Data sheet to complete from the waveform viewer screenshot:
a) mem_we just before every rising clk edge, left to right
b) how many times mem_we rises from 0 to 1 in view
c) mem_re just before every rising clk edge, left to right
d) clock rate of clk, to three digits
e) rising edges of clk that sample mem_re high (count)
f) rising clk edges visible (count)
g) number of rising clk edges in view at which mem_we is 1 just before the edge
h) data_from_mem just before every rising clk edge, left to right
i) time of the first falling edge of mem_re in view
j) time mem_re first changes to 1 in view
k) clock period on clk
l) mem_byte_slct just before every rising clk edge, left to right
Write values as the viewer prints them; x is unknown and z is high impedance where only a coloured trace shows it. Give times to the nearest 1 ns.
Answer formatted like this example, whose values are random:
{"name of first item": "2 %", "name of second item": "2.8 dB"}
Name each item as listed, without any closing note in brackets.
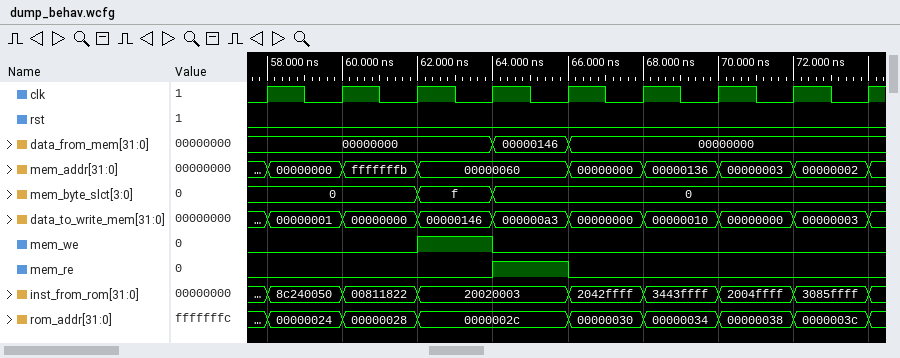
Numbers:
{"mem_we just before every rising clk edge, left to right": "0 0 0 1 0 0 0 0 0", "how many times mem_we rises from 0 to 1 in view": "1", "mem_re just before every rising clk edge, left to right": "0 0 0 0 1 0 0 0 0", "clock rate of clk, to three digits": "500 MHz", "rising edges of clk that sample mem_re high": "1", "rising clk edges visible": "9", "number of rising clk edges in view at which mem_we is 1 just before the edge": "1", "data_from_mem just before every rising clk edge, left to right": "00000000, 00000000, 00000000, 00000000, 00000146, 00000000, 00000000, 00000000, 00000000", "time of the first falling edge of mem_re in view": "66 ns", "time mem_re first changes to 1 in view": "64 ns", "clock period on clk": "2 ns", "mem_byte_slct just before every rising clk edge, left to right": "0, 0, 0, f, 0, 0, 0, 0, 0"}
